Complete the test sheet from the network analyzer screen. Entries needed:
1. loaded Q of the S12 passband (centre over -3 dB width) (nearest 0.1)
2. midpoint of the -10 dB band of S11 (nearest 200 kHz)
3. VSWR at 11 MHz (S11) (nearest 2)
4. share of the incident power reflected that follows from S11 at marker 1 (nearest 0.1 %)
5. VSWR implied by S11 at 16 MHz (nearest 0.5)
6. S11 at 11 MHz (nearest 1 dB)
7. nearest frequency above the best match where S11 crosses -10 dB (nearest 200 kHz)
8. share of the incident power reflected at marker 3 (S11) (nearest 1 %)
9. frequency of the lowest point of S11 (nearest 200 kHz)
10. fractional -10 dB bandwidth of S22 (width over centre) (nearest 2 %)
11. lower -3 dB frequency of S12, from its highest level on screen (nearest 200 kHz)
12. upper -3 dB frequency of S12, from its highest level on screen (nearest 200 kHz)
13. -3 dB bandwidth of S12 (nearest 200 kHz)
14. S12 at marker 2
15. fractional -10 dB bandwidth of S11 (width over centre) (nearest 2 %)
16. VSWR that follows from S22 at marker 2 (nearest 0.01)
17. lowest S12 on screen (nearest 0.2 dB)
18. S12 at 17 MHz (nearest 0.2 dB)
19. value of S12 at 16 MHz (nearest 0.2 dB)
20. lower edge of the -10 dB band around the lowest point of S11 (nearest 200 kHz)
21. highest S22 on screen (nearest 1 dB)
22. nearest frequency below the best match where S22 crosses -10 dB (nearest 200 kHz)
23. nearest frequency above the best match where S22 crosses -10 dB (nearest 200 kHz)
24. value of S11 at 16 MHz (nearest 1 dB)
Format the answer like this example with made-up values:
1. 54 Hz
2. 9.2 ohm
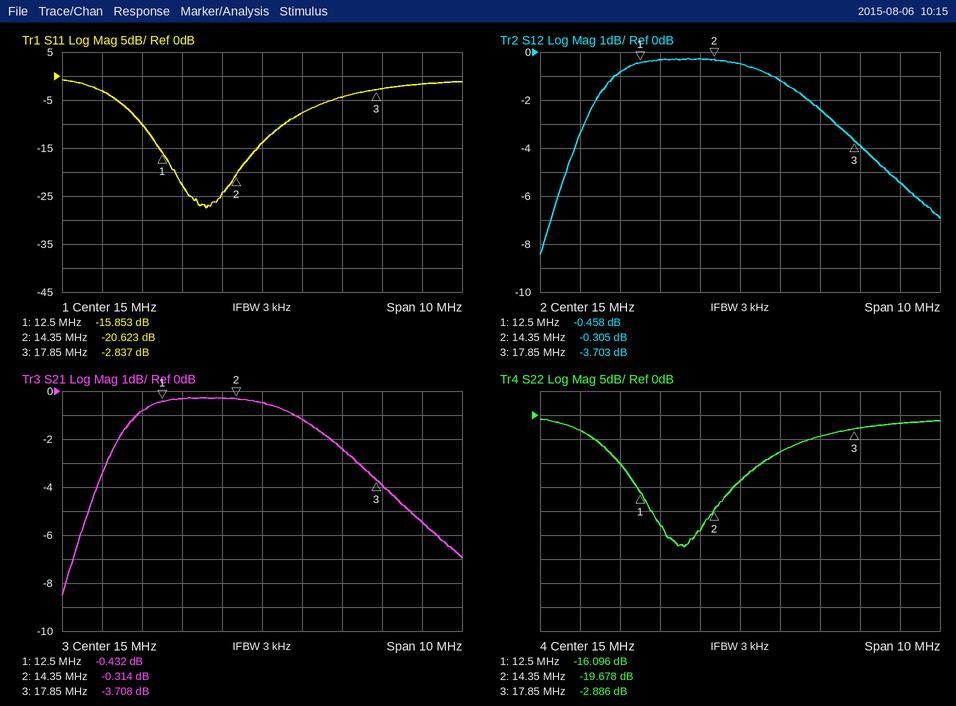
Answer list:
1. 2.2
2. 13.8 MHz
3. 6
4. 2.6 %
5. 2.5
6. -3 dB
7. 15.6 MHz
8. 52 %
9. 13.6 MHz
10. 26 %
11. 11.0 MHz
12. 17.6 MHz
13. 6.6 MHz
14. -0.305 dB
15. 26 %
16. 1.23
17. -8.4 dB
18. -2.4 dB
19. -1.2 dB
20. 12.0 MHz
21. -1 dB
22. 12.0 MHz
23. 15.6 MHz
24. -8 dB
